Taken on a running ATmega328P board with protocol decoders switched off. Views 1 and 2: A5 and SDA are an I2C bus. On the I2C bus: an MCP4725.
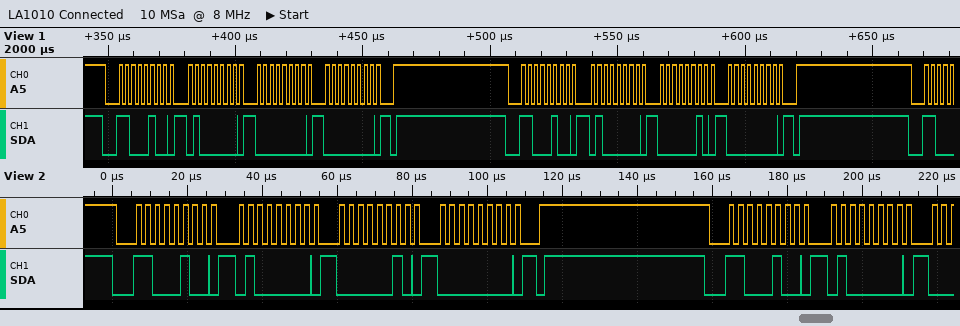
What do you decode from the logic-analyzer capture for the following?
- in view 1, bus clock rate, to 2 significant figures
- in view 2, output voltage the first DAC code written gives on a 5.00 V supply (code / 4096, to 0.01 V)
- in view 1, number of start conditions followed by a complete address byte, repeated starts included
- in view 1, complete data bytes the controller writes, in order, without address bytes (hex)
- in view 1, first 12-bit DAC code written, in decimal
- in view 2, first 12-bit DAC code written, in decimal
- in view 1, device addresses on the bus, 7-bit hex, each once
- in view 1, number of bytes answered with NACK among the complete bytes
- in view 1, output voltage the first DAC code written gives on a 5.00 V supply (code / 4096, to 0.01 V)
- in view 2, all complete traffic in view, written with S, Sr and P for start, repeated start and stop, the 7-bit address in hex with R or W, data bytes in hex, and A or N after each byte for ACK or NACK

400 kHz
0.04 V
2
40 00 00 40 02 00
0
32
0x62
0
0.00 V
S 62W A 40 A 02 A 00 A P S 62W A 40 A
